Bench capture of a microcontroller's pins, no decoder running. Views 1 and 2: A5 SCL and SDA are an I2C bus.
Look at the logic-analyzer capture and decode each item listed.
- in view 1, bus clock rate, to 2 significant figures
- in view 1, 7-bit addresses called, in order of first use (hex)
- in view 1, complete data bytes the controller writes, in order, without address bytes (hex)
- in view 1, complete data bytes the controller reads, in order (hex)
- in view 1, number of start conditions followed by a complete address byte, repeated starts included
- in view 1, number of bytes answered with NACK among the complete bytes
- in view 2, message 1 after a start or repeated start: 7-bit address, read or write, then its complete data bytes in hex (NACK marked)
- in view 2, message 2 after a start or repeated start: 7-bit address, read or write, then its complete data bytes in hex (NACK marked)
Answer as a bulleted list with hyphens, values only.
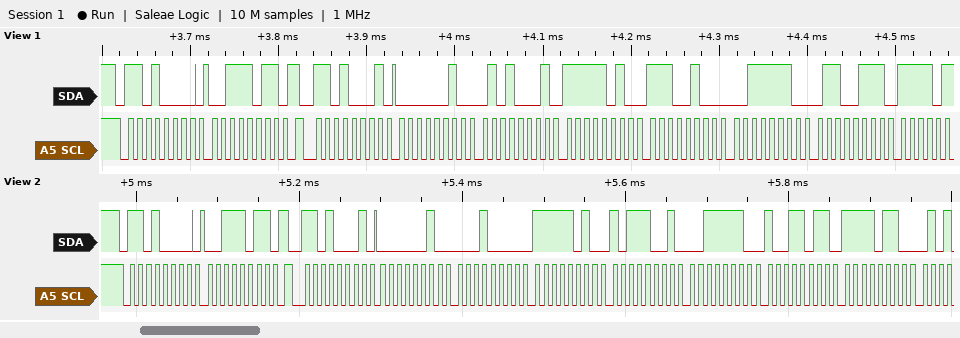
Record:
- 100 kHz
- 0x68
- 3B
- 02 51 FA E4 3E 67
- 2
- 0
- 0x68 write: 3B
- 0x68 read: 02 10 FA B9 3E 9B F6
